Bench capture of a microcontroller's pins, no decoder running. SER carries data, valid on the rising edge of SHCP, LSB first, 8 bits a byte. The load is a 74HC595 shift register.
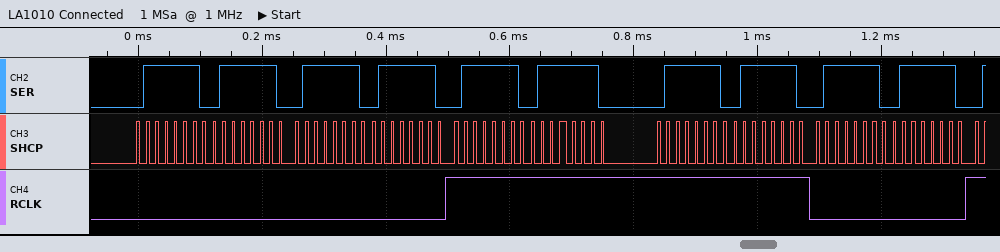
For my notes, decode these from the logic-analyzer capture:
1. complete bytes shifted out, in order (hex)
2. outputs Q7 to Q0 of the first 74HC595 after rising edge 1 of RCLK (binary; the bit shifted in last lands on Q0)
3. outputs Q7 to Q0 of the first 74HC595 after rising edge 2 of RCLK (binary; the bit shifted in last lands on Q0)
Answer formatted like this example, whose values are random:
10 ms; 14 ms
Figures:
7E 7E 7E 7E 7E 7E 7E 7E 7E 7E; 01111110; 01111110
